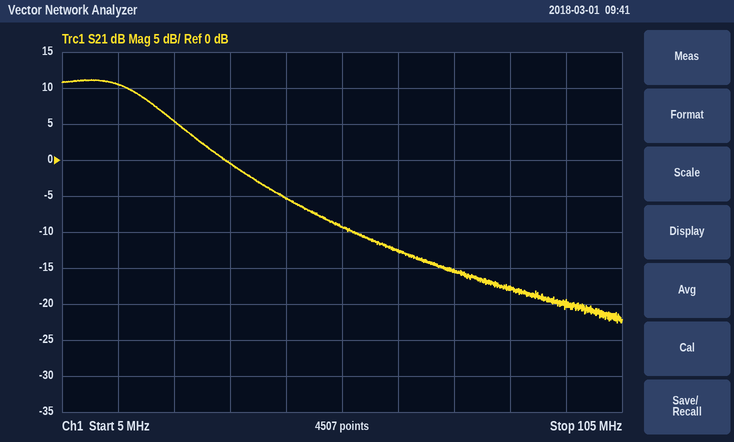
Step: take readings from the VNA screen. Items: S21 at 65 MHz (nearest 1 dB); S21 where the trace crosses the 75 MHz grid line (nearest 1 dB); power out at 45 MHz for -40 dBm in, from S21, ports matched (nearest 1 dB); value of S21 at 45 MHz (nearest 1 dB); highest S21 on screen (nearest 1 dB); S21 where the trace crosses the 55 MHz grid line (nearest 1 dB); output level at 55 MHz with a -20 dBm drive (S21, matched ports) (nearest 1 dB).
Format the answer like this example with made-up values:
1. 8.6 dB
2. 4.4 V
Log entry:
1. -13 dB
2. -15 dB
3. -45 dBm
4. -5 dB
5. 11 dB
6. -9 dB
7. -29 dBm
